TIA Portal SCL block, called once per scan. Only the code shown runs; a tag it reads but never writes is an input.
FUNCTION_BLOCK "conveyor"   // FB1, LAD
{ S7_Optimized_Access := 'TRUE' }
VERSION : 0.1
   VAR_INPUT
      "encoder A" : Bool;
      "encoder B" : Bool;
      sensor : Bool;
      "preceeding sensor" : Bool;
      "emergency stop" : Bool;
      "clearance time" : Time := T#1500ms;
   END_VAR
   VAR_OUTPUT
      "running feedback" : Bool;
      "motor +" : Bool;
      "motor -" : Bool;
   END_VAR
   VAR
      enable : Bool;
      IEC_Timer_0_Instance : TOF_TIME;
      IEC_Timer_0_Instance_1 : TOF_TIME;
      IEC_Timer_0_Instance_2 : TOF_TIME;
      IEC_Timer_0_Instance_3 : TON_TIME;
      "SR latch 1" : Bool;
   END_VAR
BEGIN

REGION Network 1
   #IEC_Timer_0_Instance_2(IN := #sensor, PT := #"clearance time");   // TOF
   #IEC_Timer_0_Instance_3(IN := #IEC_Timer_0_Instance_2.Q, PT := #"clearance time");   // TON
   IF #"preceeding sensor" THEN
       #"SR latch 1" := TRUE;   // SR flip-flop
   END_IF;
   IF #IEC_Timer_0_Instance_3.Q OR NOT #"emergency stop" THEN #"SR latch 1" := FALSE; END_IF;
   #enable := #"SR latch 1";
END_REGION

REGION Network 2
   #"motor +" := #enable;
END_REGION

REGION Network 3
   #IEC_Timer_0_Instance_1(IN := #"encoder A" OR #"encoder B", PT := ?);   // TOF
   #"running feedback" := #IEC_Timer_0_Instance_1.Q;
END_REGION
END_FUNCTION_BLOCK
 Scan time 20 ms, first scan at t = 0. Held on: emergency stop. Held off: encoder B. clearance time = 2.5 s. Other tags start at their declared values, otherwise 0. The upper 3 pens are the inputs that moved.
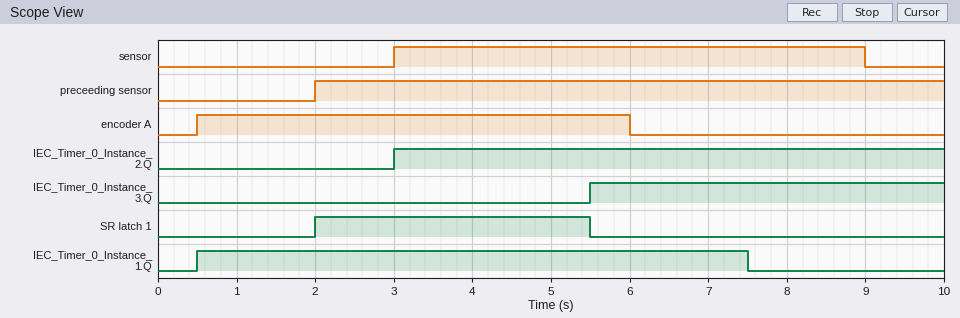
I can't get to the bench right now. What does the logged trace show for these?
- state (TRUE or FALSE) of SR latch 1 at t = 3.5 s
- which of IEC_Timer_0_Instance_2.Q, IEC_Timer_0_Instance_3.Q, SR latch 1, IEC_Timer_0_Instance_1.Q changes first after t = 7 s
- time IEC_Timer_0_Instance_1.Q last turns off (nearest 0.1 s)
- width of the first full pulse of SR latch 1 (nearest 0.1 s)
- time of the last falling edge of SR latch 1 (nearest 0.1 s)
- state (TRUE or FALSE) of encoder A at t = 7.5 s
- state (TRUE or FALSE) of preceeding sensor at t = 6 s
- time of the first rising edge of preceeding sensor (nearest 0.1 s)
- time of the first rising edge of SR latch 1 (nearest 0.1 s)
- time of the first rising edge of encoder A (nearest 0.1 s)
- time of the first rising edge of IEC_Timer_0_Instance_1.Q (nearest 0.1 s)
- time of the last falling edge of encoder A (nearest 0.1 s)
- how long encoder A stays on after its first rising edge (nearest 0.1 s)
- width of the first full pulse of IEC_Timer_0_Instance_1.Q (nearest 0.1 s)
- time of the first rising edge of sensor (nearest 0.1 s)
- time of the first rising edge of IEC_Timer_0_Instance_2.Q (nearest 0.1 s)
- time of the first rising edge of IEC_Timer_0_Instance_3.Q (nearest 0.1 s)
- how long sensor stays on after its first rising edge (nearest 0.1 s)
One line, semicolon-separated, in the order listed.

TRUE; IEC_Timer_0_Instance_1.Q; 7.5 s; 3.5 s; 5.5 s; FALSE; TRUE; 2.0 s; 2.0 s; 0.5 s; 0.5 s; 6.0 s; 5.5 s; 7.0 s; 3.0 s; 3.0 s; 5.5 s; 6.0 s
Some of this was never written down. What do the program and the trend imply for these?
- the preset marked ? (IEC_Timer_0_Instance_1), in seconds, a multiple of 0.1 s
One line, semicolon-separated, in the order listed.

1.5 s
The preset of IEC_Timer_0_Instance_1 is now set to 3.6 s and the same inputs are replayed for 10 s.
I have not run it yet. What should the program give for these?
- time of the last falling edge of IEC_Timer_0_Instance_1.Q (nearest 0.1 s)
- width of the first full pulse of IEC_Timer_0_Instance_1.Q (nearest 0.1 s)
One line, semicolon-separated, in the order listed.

9.6 s; 9.1 s
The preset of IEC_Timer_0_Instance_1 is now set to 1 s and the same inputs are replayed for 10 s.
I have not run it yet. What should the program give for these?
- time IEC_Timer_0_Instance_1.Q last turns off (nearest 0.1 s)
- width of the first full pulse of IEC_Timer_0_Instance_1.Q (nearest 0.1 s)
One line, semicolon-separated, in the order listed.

7.0 s; 6.5 s
